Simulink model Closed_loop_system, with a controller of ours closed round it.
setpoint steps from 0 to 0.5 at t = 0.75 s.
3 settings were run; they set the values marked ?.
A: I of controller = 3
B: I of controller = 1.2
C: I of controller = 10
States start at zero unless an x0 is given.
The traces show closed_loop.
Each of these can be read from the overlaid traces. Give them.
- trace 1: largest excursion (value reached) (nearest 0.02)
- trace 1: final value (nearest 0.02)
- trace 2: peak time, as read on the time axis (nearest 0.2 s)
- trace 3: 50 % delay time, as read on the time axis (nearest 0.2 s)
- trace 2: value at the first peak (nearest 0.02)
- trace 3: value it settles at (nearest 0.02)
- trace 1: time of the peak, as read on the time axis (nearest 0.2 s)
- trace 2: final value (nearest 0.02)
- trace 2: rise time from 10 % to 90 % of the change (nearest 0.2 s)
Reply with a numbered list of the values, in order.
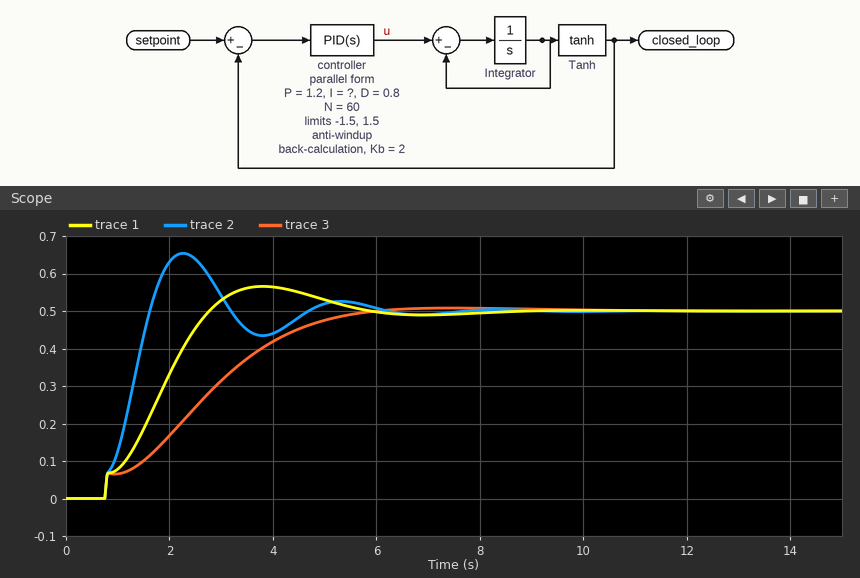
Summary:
1. 0.56
2. 0.50
3. 2.2 s
4. 2.6 s
5. 0.66
6. 0.50
7. 3.8 s
8. 0.50
9. 0.8 s
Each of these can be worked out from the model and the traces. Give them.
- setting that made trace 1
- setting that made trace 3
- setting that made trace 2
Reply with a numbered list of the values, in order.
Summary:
1. A
2. B
3. C
